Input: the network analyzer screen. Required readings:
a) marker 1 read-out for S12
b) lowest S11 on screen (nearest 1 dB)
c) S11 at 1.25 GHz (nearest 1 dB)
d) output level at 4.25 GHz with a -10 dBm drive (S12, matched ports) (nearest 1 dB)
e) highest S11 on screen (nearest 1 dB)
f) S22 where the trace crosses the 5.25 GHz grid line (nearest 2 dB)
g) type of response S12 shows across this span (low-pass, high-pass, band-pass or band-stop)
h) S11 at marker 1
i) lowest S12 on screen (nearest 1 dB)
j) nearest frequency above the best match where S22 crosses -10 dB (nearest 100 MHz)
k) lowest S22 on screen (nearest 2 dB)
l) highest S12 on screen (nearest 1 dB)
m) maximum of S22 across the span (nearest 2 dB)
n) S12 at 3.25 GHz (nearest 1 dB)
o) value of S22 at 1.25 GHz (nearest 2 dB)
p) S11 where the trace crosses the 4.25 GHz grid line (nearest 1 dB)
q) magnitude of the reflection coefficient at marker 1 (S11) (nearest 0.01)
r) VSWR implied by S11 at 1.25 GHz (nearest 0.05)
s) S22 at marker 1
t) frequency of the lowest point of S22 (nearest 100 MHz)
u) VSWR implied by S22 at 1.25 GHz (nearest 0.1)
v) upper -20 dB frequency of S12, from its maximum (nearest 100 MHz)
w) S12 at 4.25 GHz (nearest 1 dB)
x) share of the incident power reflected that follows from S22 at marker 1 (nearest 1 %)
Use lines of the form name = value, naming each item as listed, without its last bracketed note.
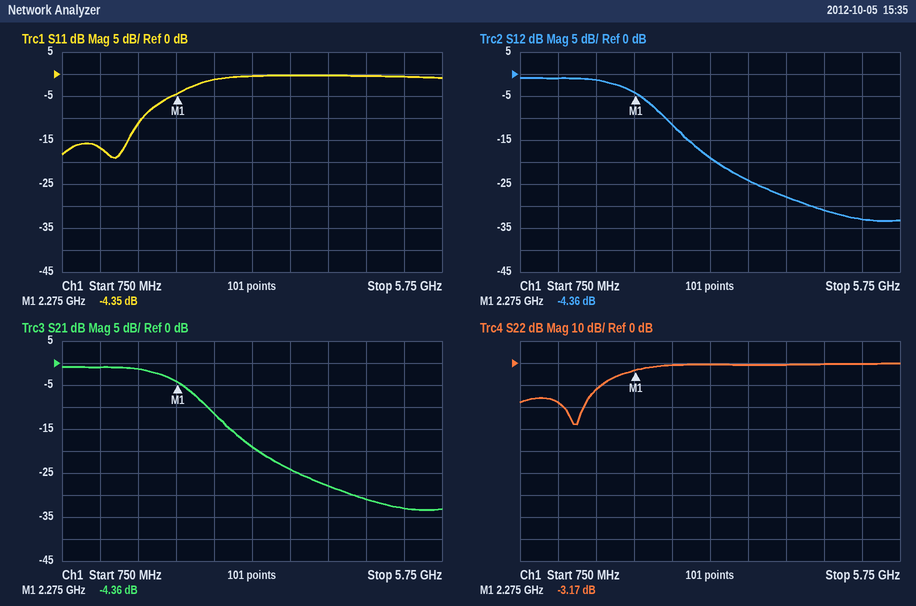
marker 1 read-out for S12 = -4.36 dB
lowest S11 on screen = -19 dB
S11 at 1.25 GHz = -17 dB
output level at 4.25 GHz with a -10 dBm drive (S12, matched ports) = -38 dBm
highest S11 on screen = 0 dB
S22 where the trace crosses the 5.25 GHz grid line = 0 dB
type of response S12 shows across this span = low-pass
S11 at marker 1 = -4.35 dB
lowest S12 on screen = -33 dB
nearest frequency above the best match where S22 crosses -10 dB = 1.8 GHz
lowest S22 on screen = -28 dB
highest S12 on screen = -1 dB
maximum of S22 across the span = 0 dB
S12 at 3.25 GHz = -19 dB
value of S22 at 1.25 GHz = -18 dB
S11 where the trace crosses the 4.25 GHz grid line = 0 dB
magnitude of the reflection coefficient at marker 1 (S11) = 0.61
VSWR implied by S11 at 1.25 GHz = 1.35
S22 at marker 1 = -3.17 dB
frequency of the lowest point of S22 = 1.5 GHz
VSWR implied by S22 at 1.25 GHz = 1.3
upper -20 dB frequency of S12, from its maximum = 3.4 GHz
S12 at 4.25 GHz = -28 dB
share of the incident power reflected that follows from S22 at marker 1 = 48 %
